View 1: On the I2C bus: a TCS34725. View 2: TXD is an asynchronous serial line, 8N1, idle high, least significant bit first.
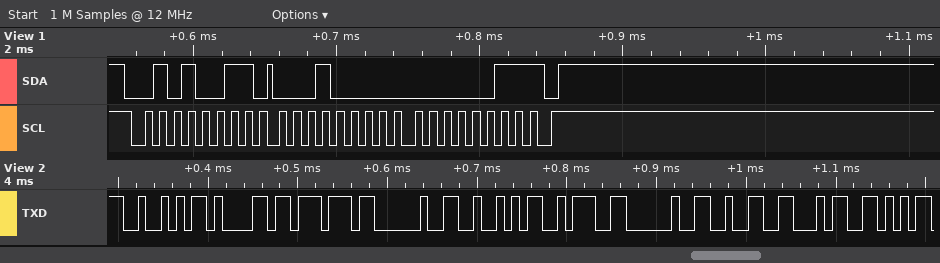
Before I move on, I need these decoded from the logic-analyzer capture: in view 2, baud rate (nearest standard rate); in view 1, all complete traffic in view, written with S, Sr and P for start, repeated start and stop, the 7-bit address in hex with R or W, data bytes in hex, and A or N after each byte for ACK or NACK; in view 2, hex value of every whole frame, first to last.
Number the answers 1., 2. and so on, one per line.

1. 115200 baud
2. S 29R A 10 A 03 N P
3. 0x52 0x61 0x77 0x20 0x52 0x3A 0x20 0x32 0x34
